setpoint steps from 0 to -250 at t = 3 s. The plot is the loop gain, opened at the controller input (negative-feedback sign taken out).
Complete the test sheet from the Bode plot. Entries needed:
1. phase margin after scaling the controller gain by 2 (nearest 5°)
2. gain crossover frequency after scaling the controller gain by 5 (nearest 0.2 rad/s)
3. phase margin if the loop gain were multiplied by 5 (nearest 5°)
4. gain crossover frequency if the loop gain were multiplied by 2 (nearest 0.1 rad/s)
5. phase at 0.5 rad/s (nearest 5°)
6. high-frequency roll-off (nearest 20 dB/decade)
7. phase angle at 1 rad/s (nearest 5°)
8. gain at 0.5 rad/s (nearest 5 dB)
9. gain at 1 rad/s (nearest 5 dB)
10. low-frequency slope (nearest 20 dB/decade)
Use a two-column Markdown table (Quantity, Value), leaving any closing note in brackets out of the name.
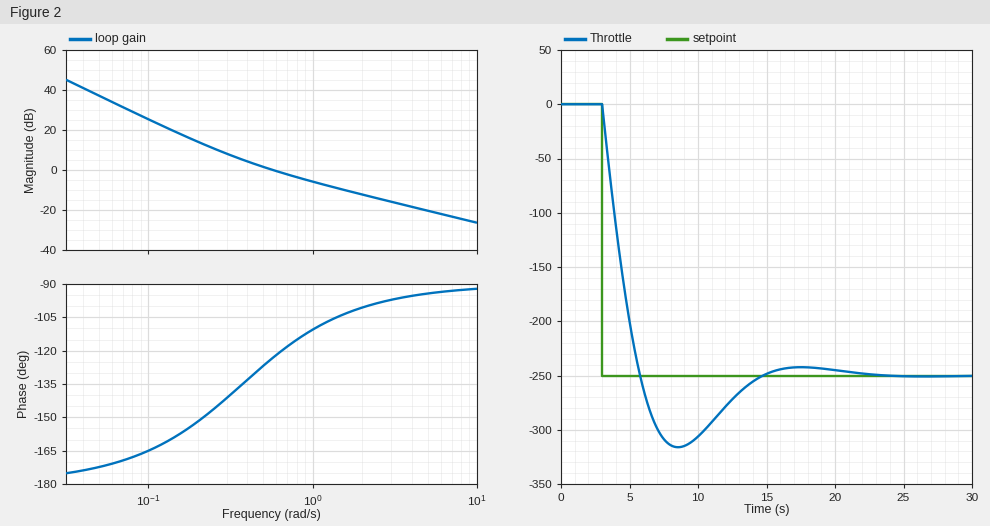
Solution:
| Quantity | Value |
|---|---|
| phase margin after scaling the controller gain by 2 | 70° |
| gain crossover frequency after scaling the controller gain by 5 | 2.4 rad/s |
| phase margin if the loop gain were multiplied by 5 | 80° |
| gain crossover frequency if the loop gain were multiplied by 2 | 1.0 rad/s |
| phase at 0.5 rad/s | -125° |
| high-frequency roll-off | -20 dB/decade |
| phase angle at 1 rad/s | -110° |
| gain at 0.5 rad/s | 0 dB |
| gain at 1 rad/s | -5 dB |
| low-frequency slope | -40 dB/decade |
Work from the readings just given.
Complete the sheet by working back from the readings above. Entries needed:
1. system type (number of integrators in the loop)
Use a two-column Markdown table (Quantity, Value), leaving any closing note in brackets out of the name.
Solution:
| Quantity | Value |
|---|---|
| system type | 2 |
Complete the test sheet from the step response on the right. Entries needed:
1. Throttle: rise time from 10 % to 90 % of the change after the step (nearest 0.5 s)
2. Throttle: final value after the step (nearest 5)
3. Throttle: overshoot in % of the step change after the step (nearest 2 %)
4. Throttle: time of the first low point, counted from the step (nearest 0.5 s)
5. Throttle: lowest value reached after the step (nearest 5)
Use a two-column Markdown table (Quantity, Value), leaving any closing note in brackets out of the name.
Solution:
| Quantity | Value |
|---|---|
| Throttle: rise time from 10 % to 90 % of the change after the step | 2.0 s |
| Throttle: final value after the step | -250 |
| Throttle: overshoot in % of the step change after the step | 26 % |
| Throttle: time of the first low point, counted from the step | 5.5 s |
| Throttle: lowest value reached after the step | -315 |
